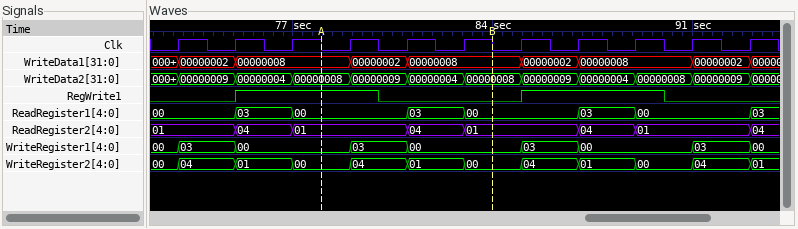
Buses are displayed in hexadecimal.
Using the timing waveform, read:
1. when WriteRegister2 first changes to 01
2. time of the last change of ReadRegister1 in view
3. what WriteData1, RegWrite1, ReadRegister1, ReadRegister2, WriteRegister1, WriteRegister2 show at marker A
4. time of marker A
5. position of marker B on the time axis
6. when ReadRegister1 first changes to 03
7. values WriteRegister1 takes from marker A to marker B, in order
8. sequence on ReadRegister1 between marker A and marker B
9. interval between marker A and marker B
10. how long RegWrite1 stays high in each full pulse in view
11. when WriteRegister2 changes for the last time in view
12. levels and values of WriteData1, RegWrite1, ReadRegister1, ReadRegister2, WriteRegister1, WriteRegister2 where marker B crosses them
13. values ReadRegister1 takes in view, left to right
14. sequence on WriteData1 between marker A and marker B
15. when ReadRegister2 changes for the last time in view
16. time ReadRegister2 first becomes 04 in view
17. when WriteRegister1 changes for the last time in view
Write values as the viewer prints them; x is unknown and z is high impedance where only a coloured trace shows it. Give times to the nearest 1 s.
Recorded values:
75 s
93 s
WriteData1=00000008, RegWrite1=1, ReadRegister1=00, ReadRegister2=01, WriteRegister1=00, WriteRegister2=00
78 s
84 s
75 s
00, 03, 00
00, 03, 00
6 s
5 s, 5 s
93 s
WriteData1=00000008, RegWrite1=0, ReadRegister1=00, ReadRegister2=01, WriteRegister1=00, WriteRegister2=00
00, 03, 00, 03, 00, 03, 00, 03
00000008, 00000002, 00000008
93 s
75 s
93 s
